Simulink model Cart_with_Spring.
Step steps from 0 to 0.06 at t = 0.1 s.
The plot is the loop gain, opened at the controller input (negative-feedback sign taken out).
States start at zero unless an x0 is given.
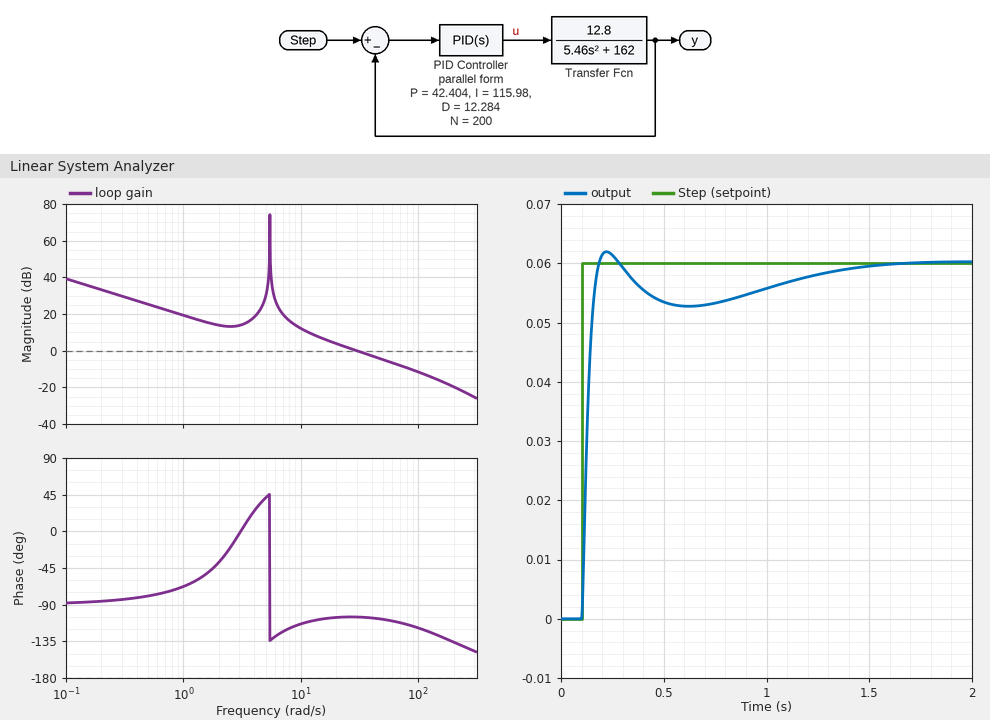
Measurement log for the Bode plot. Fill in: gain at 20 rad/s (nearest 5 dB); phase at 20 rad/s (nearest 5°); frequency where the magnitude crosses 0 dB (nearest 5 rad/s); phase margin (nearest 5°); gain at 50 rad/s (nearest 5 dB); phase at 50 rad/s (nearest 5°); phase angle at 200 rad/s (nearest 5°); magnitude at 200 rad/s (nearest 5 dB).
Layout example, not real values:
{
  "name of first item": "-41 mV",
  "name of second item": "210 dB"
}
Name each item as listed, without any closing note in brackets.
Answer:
{
  "gain at 20 rad/s": "5 dB",
  "phase at 20 rad/s": "-105°",
  "frequency where the magnitude crosses 0 dB": "30 rad/s",
  "phase margin": "75°",
  "gain at 50 rad/s": "-5 dB",
  "phase at 50 rad/s": "-110°",
  "phase angle at 200 rad/s": "-135°",
  "magnitude at 200 rad/s": "-20 dB"
}
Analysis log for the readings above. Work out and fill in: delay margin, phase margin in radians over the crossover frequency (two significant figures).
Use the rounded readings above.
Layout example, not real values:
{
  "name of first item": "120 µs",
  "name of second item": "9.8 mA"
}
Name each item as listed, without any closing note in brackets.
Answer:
{
  "delay margin, phase margin in radians over the crossover frequency": "0.044 s"
}
